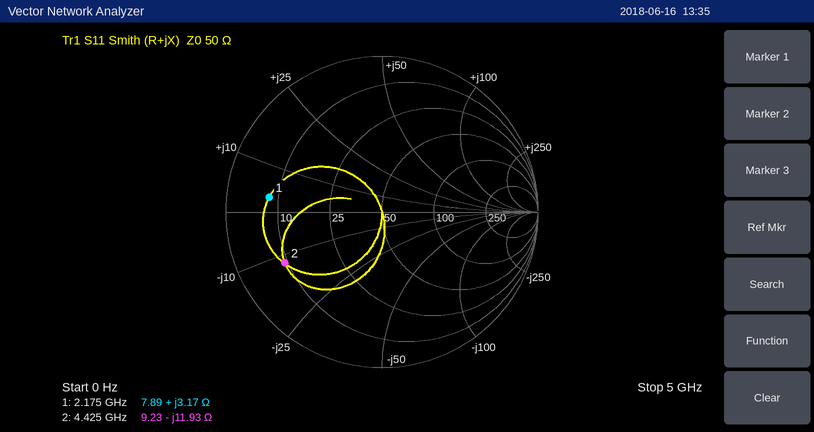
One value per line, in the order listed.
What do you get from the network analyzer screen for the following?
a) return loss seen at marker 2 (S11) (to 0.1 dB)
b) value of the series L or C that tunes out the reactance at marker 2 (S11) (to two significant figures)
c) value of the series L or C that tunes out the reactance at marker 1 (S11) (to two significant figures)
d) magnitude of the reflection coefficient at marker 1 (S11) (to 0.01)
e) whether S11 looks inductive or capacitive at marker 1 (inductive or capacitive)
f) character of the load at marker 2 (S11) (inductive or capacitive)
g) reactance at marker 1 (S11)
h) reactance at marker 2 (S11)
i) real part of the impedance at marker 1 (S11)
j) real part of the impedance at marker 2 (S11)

3.1 dB
430 pH
23 pF
0.73
inductive
capacitive
+3.17 Ω
-11.93 Ω
7.89 Ω
9.23 Ω
